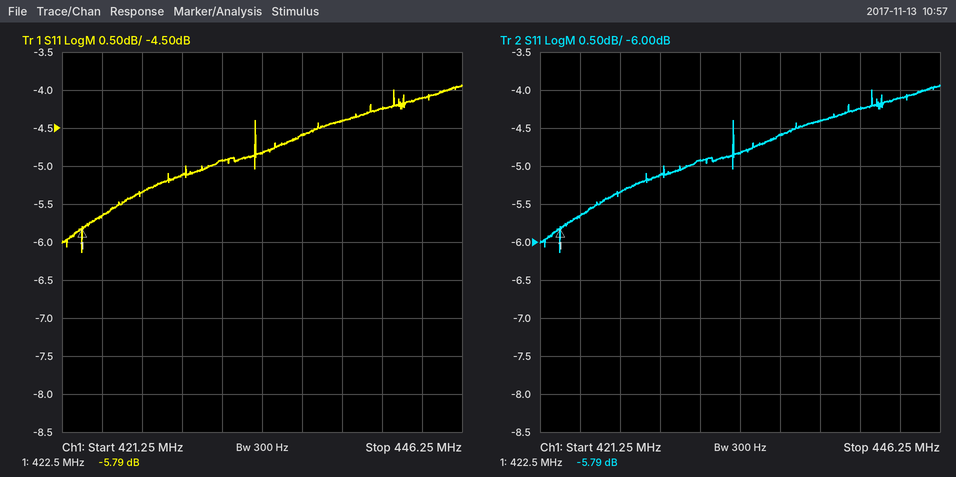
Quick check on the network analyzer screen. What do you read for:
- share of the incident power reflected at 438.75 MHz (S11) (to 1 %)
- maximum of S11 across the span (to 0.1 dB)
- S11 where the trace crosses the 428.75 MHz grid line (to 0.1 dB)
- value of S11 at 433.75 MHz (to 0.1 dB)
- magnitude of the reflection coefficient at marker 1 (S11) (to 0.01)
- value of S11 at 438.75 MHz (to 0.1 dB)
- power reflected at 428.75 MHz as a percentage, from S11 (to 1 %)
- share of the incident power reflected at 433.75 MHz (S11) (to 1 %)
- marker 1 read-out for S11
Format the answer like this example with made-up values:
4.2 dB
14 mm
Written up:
36 %
-3.9 dB
-5.1 dB
-4.8 dB
0.51
-4.4 dB
31 %
33 %
-5.79 dB
